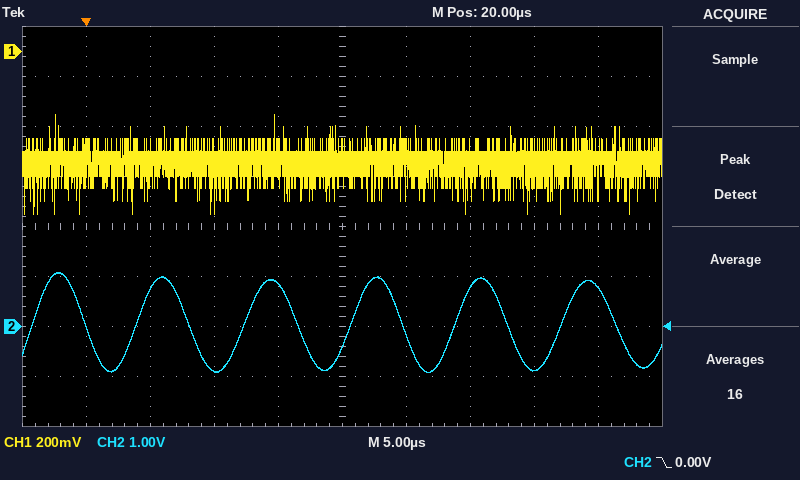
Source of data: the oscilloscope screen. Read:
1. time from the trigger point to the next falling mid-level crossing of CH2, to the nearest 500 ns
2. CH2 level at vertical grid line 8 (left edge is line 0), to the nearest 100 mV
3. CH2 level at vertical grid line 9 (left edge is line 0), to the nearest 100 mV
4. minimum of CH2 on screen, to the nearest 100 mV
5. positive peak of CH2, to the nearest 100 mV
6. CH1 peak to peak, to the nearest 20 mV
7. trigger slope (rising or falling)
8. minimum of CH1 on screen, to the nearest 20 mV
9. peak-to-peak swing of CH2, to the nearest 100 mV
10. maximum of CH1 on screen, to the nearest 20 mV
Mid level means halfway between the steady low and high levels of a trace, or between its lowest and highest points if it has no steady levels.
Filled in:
8.0 µs
-900 mV
800 mV
-900 mV
1.1 V
400 mV
falling
-660 mV
2.0 V
-260 mV
